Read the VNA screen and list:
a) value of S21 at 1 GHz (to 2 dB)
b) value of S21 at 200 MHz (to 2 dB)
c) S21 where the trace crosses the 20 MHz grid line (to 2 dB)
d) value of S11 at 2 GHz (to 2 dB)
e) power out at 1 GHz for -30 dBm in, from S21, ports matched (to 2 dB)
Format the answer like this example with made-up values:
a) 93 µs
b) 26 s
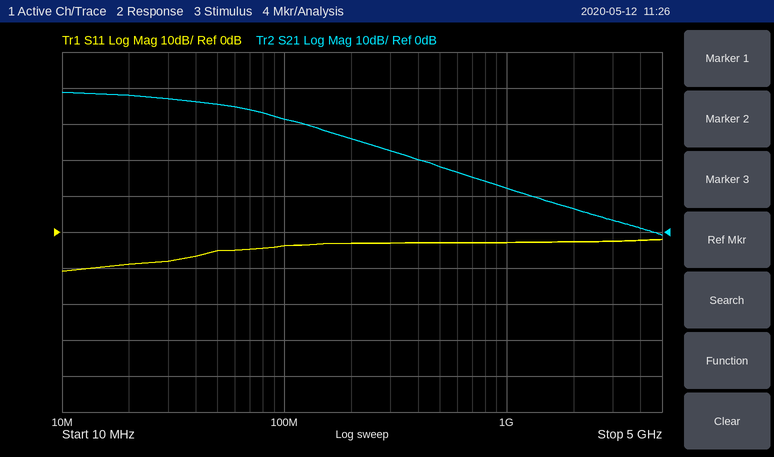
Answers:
a) 12 dB
b) 26 dB
c) 38 dB
d) -2 dB
e) -18 dBm
